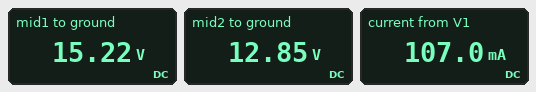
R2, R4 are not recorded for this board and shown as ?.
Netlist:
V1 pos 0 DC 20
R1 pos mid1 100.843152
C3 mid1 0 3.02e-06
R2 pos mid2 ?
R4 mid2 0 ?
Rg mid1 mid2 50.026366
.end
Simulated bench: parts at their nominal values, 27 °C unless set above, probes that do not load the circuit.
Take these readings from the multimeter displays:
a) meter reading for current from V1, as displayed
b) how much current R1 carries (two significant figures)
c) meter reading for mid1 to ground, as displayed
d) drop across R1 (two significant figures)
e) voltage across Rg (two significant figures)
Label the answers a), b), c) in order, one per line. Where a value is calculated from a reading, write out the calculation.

a) 107.0 mA
b) (20 V - 15.22 V) / 100.8 Ω = 47 mA
c) 15.22 V
d) 20 V - 15.22 V = 4.8 V
e) 15.22 V - 12.85 V = 2.4 V
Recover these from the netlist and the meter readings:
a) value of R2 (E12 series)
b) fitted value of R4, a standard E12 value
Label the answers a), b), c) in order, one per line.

a) 120 Ω
b) 120 Ω
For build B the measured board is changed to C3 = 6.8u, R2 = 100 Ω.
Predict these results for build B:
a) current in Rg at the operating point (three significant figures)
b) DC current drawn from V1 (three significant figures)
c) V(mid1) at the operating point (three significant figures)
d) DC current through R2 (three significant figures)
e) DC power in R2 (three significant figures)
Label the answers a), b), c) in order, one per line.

a) 44.3 mA
b) 111 mA
c) 15.5 V
d) 66.8 mA
e) 446 mW
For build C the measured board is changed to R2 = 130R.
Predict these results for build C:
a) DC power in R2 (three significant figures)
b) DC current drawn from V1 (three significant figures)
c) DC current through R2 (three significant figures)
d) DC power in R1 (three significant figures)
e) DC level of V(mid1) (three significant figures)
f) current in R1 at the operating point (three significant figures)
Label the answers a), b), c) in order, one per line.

a) 416 mW
b) 105 mA
c) 56.6 mA
d) 240 mW
e) 15.1 V
f) 48.8 mA
